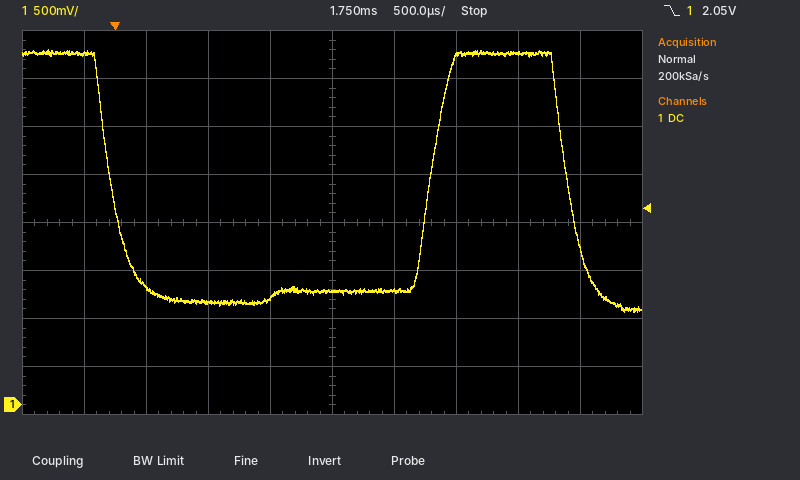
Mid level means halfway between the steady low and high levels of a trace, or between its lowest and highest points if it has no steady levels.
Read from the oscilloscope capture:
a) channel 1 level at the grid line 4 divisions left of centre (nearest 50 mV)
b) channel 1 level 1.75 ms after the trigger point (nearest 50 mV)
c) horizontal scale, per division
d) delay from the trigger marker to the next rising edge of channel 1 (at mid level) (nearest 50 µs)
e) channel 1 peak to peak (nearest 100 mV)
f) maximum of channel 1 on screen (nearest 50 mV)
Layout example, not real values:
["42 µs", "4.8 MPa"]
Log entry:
["3.65 V", "1.20 V", "500 µs", "2.55 ms", "2.70 V", "3.70 V"]
